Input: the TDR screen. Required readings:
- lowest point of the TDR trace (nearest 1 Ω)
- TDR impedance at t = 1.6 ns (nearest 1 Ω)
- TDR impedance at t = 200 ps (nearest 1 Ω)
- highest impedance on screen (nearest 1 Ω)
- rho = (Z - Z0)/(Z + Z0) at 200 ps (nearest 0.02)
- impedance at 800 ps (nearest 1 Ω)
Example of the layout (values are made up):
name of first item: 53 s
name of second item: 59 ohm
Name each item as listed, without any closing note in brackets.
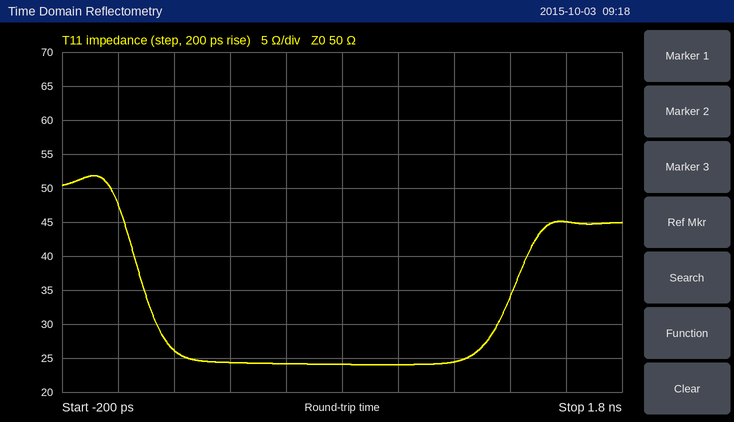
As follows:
lowest point of the TDR trace: 24 Ω
TDR impedance at t = 1.6 ns: 45 Ω
TDR impedance at t = 200 ps: 26 Ω
highest impedance on screen: 52 Ω
rho = (Z - Z0)/(Z + Z0) at 200 ps: -0.32
impedance at 800 ps: 24 Ω
